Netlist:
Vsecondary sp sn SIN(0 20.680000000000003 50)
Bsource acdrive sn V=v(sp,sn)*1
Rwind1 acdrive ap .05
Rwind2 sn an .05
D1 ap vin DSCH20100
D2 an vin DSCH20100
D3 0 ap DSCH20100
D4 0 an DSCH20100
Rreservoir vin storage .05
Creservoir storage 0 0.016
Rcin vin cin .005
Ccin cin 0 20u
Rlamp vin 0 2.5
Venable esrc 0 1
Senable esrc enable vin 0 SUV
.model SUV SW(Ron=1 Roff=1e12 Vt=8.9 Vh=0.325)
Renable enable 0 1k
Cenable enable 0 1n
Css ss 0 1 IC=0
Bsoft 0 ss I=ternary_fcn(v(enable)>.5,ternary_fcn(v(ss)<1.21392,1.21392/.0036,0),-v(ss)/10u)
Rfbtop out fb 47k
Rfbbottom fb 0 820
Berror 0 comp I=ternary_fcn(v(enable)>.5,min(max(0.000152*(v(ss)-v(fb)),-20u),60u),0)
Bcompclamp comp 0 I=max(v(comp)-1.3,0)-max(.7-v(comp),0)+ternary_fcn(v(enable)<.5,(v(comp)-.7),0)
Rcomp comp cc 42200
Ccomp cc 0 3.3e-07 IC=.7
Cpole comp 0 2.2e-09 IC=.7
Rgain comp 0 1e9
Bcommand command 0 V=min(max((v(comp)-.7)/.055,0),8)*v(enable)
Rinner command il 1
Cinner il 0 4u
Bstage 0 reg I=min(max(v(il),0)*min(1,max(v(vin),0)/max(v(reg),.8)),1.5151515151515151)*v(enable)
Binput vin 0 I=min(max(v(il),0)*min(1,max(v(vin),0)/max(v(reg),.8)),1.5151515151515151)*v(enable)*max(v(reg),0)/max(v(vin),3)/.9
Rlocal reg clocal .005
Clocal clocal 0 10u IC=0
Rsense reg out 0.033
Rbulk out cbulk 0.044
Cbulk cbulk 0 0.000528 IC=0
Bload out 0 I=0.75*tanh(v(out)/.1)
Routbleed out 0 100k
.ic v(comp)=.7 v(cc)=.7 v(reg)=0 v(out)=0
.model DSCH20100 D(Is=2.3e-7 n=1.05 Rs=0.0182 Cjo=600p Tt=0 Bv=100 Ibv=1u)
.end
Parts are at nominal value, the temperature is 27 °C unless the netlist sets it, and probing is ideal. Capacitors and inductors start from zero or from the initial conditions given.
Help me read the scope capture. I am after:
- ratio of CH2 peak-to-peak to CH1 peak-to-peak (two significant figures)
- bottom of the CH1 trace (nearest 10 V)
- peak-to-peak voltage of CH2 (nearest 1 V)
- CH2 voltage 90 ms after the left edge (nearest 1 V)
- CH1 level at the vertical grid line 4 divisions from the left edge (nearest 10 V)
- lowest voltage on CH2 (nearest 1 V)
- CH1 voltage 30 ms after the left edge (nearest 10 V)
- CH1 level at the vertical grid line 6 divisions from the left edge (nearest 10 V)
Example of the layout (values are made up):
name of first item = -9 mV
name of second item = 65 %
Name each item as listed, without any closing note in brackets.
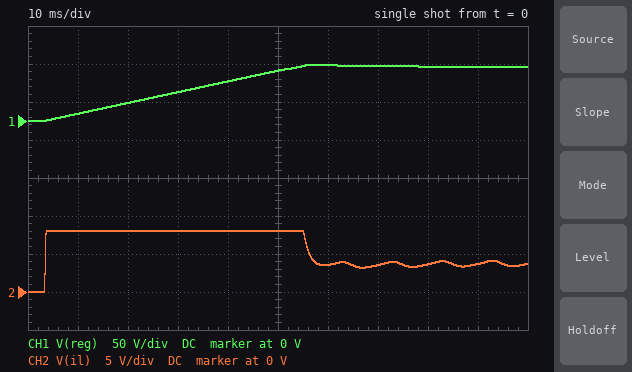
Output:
ratio of CH2 peak-to-peak to CH1 peak-to-peak = 0.11
bottom of the CH1 trace = 0 V
peak-to-peak voltage of CH2 = 8 V
CH2 voltage 90 ms after the left edge = 4 V
CH1 level at the vertical grid line 4 divisions from the left edge = 50 V
lowest voltage on CH2 = 0 V
CH1 voltage 30 ms after the left edge = 40 V
CH1 level at the vertical grid line 6 divisions from the left edge = 70 V
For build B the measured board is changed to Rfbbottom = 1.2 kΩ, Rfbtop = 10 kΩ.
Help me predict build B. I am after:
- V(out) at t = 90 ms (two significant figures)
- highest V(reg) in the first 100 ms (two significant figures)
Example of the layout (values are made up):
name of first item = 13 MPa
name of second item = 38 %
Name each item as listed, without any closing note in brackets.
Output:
V(out) at t = 90 ms = 11 V
highest V(reg) in the first 100 ms = 12 V
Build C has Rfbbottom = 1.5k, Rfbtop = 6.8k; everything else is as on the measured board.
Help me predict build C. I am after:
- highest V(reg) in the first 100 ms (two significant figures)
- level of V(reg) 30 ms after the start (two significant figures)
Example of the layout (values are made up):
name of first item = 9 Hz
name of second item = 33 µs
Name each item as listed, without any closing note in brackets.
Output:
highest V(reg) in the first 100 ms = 7.0 V
level of V(reg) 30 ms after the start = 6.8 V
